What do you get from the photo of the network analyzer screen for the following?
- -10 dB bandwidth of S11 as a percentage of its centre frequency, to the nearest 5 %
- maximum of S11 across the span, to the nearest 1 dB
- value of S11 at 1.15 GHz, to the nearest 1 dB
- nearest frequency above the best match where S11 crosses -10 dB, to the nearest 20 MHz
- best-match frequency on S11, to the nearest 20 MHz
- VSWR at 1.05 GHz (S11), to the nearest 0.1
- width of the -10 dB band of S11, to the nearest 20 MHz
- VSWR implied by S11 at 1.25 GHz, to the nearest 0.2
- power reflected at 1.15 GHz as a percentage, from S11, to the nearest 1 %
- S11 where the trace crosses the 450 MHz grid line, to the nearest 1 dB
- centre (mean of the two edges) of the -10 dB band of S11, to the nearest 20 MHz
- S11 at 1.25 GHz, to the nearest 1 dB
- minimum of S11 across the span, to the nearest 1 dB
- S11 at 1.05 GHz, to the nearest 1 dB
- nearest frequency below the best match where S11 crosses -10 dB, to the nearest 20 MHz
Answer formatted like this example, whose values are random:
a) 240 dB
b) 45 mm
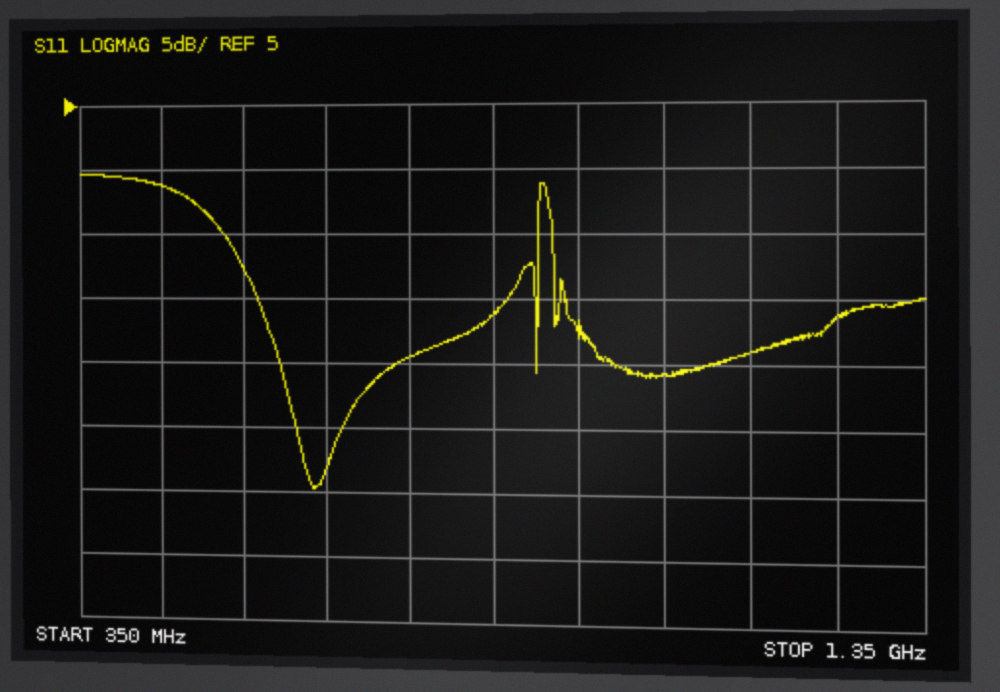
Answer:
a) 40 %
b) 0 dB
c) -14 dB
d) 860 MHz
e) 640 MHz
f) 1.4
g) 300 MHz
h) 1.8
i) 4 %
j) -1 dB
k) 720 MHz
l) -11 dB
m) -25 dB
n) -16 dB
o) 560 MHz
